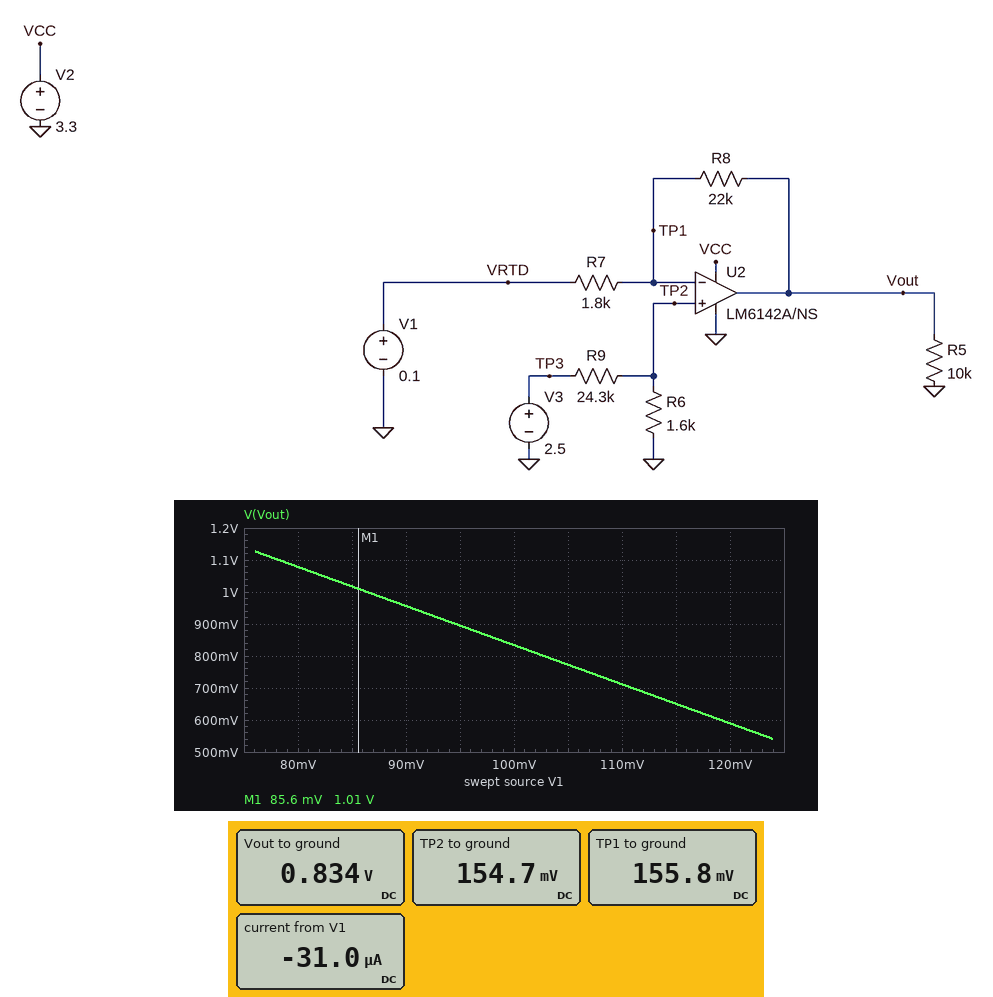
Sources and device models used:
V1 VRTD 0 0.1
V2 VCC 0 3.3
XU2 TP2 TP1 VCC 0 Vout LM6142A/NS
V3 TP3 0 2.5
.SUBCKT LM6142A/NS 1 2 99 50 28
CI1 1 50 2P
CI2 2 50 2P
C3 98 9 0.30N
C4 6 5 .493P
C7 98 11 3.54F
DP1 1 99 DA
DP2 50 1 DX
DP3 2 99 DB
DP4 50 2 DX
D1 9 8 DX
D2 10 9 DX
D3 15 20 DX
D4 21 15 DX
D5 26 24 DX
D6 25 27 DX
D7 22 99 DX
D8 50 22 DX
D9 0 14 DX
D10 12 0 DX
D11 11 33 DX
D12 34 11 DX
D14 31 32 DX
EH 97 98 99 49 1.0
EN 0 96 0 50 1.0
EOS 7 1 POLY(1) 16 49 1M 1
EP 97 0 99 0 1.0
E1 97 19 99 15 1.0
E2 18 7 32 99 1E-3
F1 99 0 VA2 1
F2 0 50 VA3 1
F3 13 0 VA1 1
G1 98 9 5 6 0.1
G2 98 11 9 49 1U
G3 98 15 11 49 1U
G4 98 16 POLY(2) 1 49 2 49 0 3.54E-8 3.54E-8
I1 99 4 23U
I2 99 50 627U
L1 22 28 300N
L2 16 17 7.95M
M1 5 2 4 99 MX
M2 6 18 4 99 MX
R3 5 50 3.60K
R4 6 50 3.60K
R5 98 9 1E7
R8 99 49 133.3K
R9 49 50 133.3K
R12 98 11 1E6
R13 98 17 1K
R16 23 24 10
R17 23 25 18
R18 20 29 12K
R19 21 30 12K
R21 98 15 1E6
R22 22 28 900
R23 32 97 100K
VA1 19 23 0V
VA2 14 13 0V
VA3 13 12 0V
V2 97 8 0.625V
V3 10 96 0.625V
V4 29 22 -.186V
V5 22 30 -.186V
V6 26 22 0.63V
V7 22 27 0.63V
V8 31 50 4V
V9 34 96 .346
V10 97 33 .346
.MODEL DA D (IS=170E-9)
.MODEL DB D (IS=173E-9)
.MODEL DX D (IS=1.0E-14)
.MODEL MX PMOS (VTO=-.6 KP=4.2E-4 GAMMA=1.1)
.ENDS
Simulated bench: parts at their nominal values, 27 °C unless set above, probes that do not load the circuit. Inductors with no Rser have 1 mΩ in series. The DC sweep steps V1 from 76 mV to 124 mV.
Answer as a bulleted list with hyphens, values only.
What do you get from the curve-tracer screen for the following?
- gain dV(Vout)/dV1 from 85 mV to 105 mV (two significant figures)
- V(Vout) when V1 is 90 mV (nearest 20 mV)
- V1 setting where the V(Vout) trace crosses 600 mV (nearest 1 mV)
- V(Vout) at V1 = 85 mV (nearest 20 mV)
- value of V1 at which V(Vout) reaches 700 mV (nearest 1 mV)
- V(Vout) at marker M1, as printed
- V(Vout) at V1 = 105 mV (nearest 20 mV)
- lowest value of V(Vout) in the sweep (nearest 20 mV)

- -12 V/V
- 960 mV
- 119 mV
- 1.02 V
- 111 mV
- 1.01 V
- 780 mV
- 540 mV
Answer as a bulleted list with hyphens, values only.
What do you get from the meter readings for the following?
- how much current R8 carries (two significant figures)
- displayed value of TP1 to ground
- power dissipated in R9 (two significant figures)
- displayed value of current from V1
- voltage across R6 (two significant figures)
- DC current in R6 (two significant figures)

- 31 µA
- 155.8 mV
- 230 µW
- -31.0 µA
- 150 mV
- 97 µA
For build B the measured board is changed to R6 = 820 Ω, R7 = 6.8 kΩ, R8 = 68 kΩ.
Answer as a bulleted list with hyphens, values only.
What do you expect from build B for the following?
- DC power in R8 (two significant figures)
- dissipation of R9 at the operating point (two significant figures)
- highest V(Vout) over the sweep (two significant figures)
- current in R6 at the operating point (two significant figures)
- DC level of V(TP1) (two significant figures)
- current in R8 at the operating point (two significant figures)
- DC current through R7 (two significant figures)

- 120 nW
- 240 µW
- 140 mV
- 100 µA
- 92 mV
- 1.3 µA
- 1.1 µA
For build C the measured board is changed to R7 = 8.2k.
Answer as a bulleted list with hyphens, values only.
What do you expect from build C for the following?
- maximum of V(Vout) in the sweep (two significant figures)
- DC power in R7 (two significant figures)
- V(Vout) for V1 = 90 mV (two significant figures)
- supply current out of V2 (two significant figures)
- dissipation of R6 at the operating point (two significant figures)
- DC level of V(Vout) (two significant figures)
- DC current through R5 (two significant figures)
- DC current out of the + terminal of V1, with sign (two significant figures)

- 370 mV
- 380 nW
- 330 mV
- 700 µA
- 15 µW
- 300 mV
- 30 µA
- -6.8 µA
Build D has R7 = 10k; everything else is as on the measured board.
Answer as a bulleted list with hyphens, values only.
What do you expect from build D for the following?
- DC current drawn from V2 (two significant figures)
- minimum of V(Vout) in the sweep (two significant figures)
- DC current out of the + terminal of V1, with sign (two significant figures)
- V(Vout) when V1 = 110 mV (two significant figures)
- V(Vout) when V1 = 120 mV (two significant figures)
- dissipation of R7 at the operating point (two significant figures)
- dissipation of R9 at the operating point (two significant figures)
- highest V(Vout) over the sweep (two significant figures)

- 700 µA
- 220 mV
- -5.6 µA
- 250 mV
- 230 mV
- 310 nW
- 230 µW
- 330 mV
